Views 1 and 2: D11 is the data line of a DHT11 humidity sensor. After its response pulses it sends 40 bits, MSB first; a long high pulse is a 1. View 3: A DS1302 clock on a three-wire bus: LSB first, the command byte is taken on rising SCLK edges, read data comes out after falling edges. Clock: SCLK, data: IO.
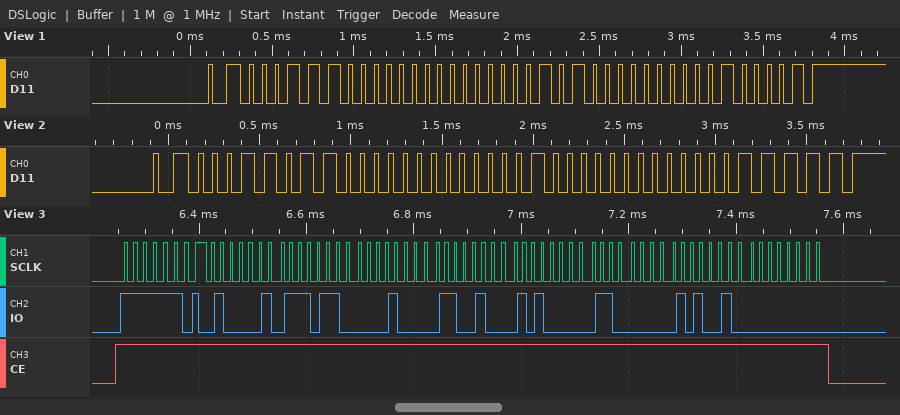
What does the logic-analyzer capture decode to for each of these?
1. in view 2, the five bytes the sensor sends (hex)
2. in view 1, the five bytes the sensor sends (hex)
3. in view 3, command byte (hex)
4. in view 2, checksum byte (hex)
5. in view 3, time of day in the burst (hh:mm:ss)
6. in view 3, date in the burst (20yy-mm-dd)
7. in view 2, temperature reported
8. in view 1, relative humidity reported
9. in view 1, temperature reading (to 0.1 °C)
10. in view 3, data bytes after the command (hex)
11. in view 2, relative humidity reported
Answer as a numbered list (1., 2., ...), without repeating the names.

1. 1B 00 04 00 1F
2. 1C 00 05 00 21
3. 0xBF
4. 0x1F
5. 08:37:42
6. 2025-05-13
7. 4.0 °C
8. 28 %
9. 5.0 °C
10. 42 37 08 13 05 03 25 00
11. 27 %
